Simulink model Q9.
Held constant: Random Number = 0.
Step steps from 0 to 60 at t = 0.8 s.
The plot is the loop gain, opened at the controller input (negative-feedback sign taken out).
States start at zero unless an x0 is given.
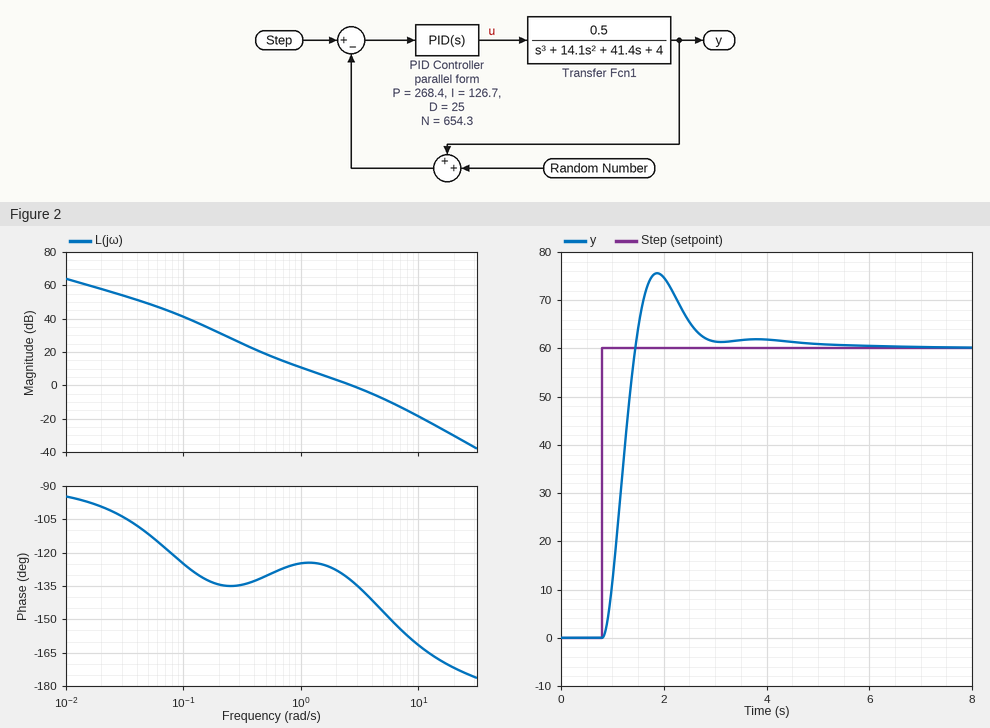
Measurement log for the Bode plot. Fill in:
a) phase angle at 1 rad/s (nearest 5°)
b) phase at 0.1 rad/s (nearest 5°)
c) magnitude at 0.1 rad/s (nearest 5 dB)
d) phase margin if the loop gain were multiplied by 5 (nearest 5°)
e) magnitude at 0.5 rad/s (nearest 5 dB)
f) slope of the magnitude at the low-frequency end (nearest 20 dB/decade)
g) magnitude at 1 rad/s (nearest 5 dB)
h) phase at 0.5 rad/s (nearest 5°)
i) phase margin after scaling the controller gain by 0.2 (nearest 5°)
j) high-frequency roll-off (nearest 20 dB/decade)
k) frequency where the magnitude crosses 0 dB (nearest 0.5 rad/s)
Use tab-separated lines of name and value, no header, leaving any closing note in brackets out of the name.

phase angle at 1 rad/s	-125°
phase at 0.1 rad/s	-125°
magnitude at 0.1 rad/s	40 dB
phase margin if the loop gain were multiplied by 5	25°
magnitude at 0.5 rad/s	20 dB
slope of the magnitude at the low-frequency end	-20 dB/decade
magnitude at 1 rad/s	10 dB
phase at 0.5 rad/s	-130°
phase margin after scaling the controller gain by 0.2	55°
high-frequency roll-off	-40 dB/decade
frequency where the magnitude crosses 0 dB	2.5 rad/s
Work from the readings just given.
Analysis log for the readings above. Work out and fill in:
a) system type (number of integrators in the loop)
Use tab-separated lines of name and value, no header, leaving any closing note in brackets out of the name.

system type	1
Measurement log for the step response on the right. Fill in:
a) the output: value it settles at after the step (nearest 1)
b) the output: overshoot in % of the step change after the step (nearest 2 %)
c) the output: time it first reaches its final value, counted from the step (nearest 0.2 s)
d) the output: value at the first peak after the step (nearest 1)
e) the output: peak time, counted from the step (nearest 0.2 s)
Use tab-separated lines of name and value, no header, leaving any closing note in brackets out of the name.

the output: value it settles at after the step	60
the output: overshoot in % of the step change after the step	26 %
the output: time it first reaches its final value, counted from the step	0.6 s
the output: value at the first peak after the step	76
the output: peak time, counted from the step	1.0 s
